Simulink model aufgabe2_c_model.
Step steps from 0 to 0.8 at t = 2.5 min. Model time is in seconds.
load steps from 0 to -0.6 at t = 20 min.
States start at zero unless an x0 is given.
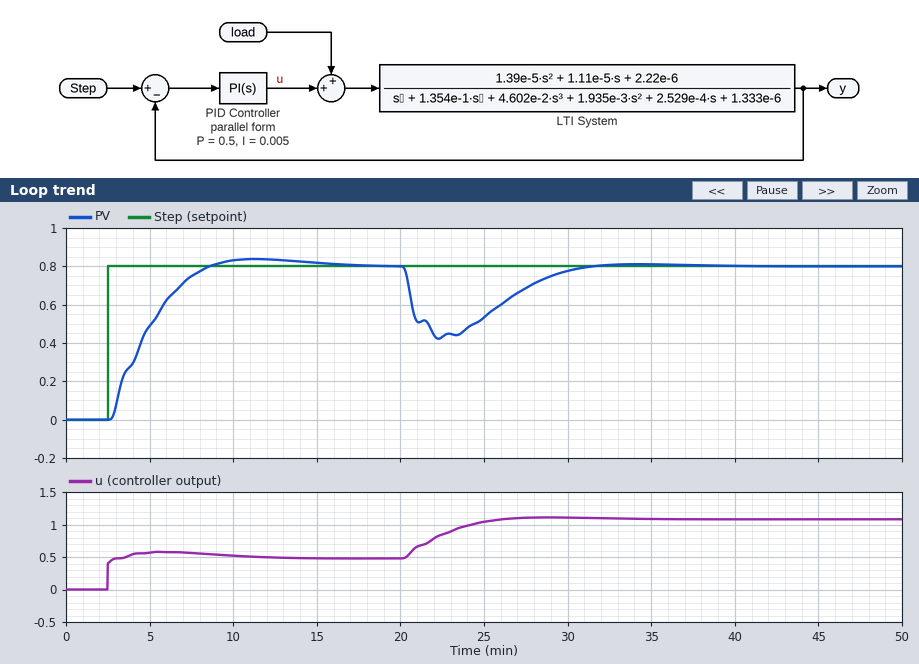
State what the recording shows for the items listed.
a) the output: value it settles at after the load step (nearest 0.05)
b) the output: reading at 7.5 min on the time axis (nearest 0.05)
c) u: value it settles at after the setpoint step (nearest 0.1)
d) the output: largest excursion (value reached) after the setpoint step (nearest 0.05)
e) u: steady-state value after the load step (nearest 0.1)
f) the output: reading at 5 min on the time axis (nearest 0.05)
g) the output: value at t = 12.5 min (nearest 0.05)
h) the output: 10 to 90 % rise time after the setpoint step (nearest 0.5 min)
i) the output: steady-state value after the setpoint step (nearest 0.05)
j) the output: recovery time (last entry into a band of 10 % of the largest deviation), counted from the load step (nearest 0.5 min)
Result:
0.80
0.75
0.5
0.85
1.1
0.50
0.85
4.0 min
0.80
9.5 min
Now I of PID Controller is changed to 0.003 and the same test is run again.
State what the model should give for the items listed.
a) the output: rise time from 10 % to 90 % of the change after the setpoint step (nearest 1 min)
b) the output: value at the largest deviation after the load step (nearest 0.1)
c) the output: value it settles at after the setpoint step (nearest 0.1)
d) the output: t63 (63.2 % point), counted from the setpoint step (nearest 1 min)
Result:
7 min
0.4
0.8
3 min
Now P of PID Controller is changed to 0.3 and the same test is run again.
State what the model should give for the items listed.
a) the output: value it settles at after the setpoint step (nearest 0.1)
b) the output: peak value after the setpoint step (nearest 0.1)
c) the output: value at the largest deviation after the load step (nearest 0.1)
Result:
0.8
0.9
0.4
